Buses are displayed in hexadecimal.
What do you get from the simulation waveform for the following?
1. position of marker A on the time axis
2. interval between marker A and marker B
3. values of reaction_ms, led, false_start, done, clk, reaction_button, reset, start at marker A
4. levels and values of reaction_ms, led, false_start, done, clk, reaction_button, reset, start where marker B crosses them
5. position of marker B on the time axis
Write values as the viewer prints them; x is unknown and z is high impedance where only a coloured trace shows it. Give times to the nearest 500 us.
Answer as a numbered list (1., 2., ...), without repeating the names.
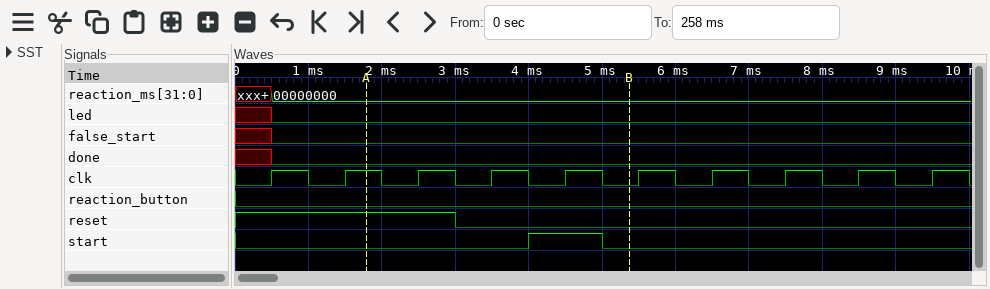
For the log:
1. 2000 us
2. 3500 us
3. reaction_ms=00000000, led=0, false_start=0, done=0, clk=1, reaction_button=0, reset=1, start=0
4. reaction_ms=00000000, led=0, false_start=0, done=0, clk=0, reaction_button=0, reset=0, start=0
5. 5500 us
